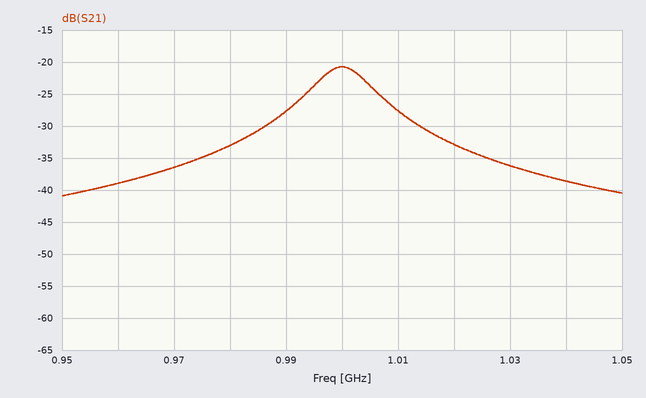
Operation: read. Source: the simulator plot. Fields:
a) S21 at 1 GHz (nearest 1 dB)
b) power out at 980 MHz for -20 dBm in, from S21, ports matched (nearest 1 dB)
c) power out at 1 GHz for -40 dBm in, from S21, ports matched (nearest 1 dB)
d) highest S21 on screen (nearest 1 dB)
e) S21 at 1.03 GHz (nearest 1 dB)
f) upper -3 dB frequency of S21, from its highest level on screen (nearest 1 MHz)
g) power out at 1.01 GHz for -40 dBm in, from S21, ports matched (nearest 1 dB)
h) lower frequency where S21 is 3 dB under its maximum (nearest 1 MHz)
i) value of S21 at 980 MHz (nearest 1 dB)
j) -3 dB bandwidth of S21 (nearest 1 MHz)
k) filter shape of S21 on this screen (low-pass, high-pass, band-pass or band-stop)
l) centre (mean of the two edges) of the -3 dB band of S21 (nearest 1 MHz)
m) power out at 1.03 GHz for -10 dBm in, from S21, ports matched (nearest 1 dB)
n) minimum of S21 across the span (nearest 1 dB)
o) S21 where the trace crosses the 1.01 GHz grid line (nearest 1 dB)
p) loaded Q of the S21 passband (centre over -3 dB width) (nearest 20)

-21 dB
-53 dBm
-61 dBm
-21 dB
-36 dB
1.005 GHz
-68 dBm
995 MHz
-33 dB
10 MHz
band-pass
1.000 GHz
-46 dBm
-41 dB
-28 dB
100
